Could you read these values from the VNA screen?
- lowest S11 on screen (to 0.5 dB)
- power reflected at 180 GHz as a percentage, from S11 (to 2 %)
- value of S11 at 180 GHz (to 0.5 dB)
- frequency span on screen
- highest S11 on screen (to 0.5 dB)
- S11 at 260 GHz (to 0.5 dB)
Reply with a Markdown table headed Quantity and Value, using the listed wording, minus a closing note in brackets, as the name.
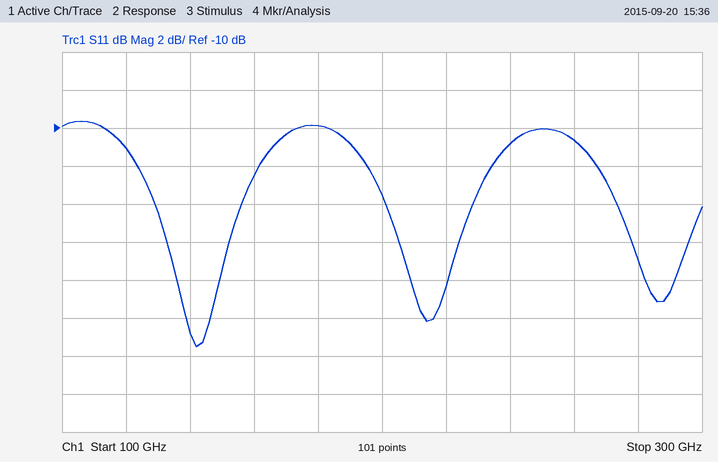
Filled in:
| Quantity | Value |
|---|---|
| lowest S11 on screen | -21.5 dB |
| power reflected at 180 GHz as a percentage, from S11 | 10 % |
| value of S11 at 180 GHz | -10.0 dB |
| frequency span on screen | 200 GHz |
| highest S11 on screen | -9.5 dB |
| S11 at 260 GHz | -10.5 dB |
